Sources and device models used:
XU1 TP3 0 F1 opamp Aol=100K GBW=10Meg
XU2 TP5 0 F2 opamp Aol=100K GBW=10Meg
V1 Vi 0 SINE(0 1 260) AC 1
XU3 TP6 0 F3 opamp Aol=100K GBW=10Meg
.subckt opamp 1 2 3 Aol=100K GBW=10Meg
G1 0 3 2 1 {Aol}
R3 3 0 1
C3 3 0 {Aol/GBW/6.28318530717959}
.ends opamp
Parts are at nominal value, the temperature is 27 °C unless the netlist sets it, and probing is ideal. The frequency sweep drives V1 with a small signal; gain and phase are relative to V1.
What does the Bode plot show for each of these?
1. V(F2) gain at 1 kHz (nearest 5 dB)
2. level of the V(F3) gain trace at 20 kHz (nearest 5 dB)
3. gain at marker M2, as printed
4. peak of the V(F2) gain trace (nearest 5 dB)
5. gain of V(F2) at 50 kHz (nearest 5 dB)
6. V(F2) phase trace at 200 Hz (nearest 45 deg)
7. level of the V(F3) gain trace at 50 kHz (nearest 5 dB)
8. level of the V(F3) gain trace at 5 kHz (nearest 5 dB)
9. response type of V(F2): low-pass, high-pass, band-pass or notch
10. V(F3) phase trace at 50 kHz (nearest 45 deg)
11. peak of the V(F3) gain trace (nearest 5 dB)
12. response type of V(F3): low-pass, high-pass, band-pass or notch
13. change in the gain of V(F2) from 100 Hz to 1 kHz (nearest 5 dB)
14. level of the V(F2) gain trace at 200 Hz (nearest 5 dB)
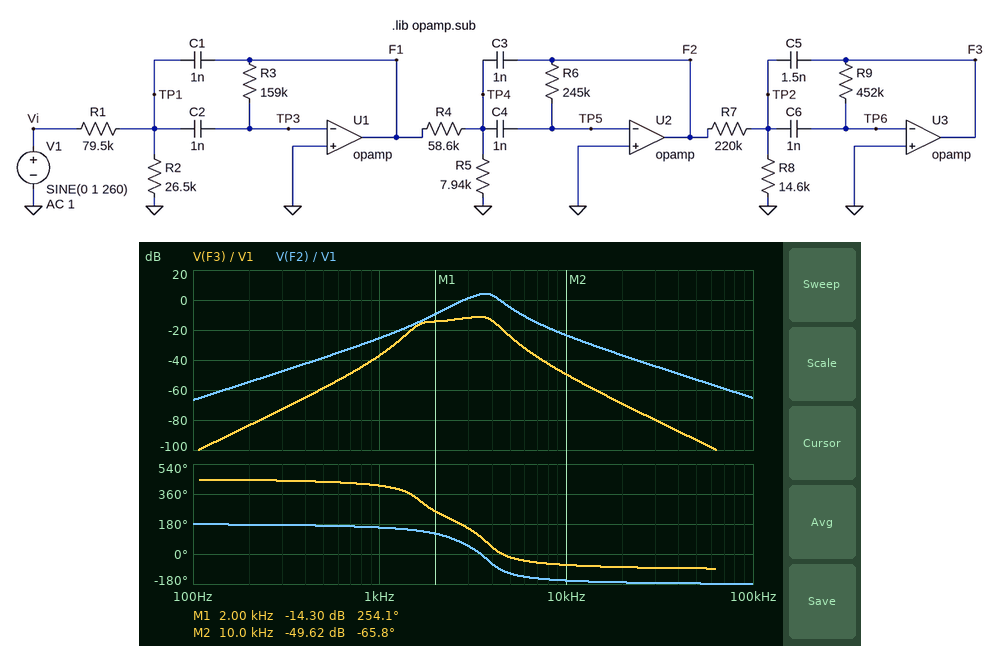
-25 dB
-70 dB
-49.62 dB
5 dB
-55 dB
180 deg
-95 dB
-25 dB
band-pass
-90 deg
-10 dB
band-pass
40 dB
-55 dB
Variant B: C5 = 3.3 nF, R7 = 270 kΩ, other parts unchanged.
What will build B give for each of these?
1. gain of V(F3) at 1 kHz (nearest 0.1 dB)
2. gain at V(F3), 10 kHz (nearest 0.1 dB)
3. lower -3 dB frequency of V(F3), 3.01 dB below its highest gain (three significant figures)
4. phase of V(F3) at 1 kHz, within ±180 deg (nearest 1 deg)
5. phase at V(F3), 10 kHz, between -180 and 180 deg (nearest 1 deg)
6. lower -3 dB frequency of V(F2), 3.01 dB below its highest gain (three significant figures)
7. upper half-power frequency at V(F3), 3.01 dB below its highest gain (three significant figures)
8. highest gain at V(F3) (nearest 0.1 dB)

-34.5 dB
-58.4 dB
2.53 kHz
5 deg
-67 deg
2.99 kHz
4.10 kHz
-21.1 dB
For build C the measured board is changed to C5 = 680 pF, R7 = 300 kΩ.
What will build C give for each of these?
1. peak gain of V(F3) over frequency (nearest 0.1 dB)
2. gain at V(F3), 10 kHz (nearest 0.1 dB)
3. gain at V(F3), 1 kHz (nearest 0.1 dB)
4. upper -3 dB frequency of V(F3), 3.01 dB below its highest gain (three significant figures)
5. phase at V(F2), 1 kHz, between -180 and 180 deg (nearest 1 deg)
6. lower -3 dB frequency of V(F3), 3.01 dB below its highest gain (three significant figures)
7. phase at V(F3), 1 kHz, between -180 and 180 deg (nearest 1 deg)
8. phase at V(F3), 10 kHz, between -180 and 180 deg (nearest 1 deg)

-3.3 dB
-45.2 dB
-41.5 dB
3.87 kHz
159 deg
2.32 kHz
59 deg
-64 deg
